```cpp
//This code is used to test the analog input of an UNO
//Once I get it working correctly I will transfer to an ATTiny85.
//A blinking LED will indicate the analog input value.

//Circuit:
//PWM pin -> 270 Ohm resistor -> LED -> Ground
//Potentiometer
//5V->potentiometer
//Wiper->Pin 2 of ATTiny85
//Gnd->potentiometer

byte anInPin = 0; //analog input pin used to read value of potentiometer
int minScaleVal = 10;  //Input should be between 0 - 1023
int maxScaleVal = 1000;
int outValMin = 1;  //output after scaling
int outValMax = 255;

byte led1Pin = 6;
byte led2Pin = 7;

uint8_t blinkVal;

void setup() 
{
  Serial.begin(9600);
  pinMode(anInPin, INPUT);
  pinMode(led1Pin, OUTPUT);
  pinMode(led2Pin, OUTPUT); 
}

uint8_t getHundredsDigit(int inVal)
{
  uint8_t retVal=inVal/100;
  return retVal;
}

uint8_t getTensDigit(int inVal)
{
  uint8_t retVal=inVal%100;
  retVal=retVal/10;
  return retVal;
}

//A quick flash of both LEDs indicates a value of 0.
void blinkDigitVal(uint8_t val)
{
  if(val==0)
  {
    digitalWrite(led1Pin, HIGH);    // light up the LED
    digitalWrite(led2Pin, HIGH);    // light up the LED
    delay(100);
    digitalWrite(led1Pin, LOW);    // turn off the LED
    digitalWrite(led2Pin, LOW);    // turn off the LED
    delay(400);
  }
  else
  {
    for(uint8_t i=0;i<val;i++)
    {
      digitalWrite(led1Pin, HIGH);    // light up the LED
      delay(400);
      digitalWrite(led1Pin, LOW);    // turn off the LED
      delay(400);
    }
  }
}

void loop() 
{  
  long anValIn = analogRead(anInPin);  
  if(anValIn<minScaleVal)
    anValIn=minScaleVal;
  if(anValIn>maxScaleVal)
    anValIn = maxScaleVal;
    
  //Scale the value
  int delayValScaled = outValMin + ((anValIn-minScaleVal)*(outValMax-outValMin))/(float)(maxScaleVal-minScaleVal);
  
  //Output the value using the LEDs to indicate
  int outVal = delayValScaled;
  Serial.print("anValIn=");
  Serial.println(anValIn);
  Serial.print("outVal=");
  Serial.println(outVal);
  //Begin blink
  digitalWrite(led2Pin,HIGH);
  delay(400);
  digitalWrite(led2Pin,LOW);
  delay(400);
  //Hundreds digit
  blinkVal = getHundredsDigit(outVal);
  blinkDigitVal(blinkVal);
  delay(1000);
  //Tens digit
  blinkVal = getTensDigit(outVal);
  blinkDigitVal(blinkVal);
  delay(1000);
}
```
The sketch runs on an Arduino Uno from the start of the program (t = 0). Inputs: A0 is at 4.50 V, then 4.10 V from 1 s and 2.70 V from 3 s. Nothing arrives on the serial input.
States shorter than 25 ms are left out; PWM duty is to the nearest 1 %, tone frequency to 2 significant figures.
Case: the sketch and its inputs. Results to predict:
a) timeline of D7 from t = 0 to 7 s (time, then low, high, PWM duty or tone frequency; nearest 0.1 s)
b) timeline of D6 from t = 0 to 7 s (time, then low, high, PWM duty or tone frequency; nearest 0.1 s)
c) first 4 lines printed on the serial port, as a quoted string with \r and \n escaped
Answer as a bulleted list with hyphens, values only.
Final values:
- 0 s high; 0.4 s low; 6.8 s high
- 0 s low; 0.8 s high; 1.2 s low; 1.6 s high; 2 s low; 3.4 s high; 3.8 s low; 4.2 s high; 4.6 s low; 5 s high; 5.4 s low
- "anValIn=921\r\noutVal=234\r\nanValIn=552\r\noutVal=140\r\n"
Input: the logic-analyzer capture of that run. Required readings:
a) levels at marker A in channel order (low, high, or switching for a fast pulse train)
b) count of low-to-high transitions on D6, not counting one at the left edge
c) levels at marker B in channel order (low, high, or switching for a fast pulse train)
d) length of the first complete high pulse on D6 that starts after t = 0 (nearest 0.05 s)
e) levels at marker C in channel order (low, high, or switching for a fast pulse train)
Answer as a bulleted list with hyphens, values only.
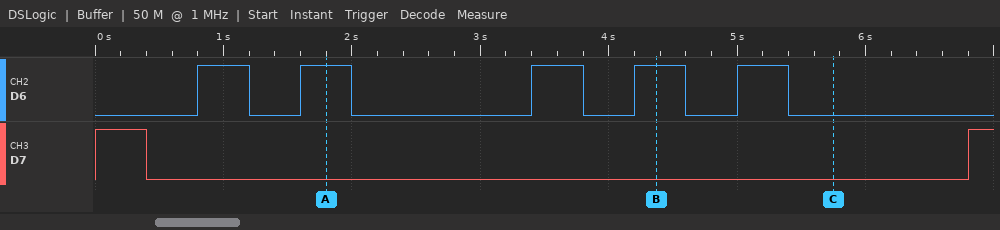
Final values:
- D6 high, D7 low
- 5
- D6 high, D7 low
- 0.40 s
- D6 low, D7 low
